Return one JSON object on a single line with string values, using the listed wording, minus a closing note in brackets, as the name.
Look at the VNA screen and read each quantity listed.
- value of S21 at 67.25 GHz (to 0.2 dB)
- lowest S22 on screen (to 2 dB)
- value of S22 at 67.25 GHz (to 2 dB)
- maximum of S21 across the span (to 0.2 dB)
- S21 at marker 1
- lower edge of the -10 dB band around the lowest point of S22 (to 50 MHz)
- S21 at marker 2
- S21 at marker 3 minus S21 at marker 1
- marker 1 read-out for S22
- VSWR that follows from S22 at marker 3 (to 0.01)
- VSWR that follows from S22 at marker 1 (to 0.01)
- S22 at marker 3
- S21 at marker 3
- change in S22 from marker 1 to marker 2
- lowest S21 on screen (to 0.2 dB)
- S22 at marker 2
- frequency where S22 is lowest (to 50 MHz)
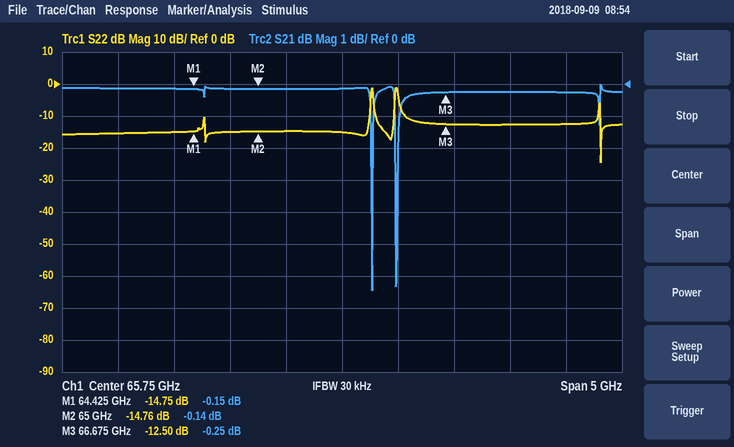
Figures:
{"value of S21 at 67.25 GHz": "-0.2 dB", "lowest S22 on screen": "-24 dB", "value of S22 at 67.25 GHz": "-12 dB", "maximum of S21 across the span": "0.0 dB", "S21 at marker 1": "-0.15 dB", "lower edge of the -10 dB band around the lowest point of S22": "68.05 GHz", "S21 at marker 2": "-0.14 dB", "S21 at marker 3 minus S21 at marker 1": "-0.10 dB", "marker 1 read-out for S22": "-14.75 dB", "VSWR that follows from S22 at marker 3": "1.62", "VSWR that follows from S22 at marker 1": "1.45", "S22 at marker 3": "-12.50 dB", "S21 at marker 3": "-0.25 dB", "change in S22 from marker 1 to marker 2": "-0.01 dB", "lowest S21 on screen": "-6.4 dB", "S22 at marker 2": "-14.76 dB", "frequency where S22 is lowest": "68.05 GHz"}
